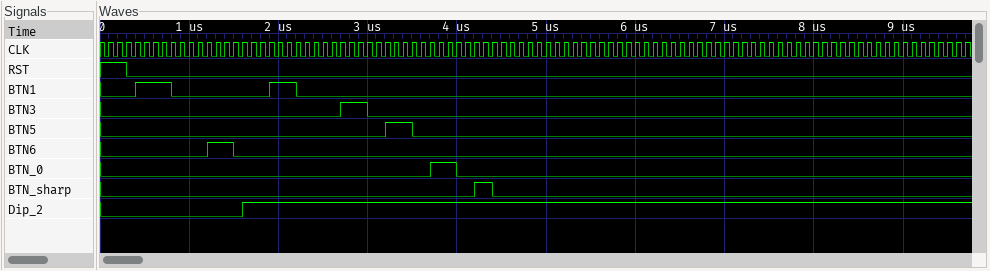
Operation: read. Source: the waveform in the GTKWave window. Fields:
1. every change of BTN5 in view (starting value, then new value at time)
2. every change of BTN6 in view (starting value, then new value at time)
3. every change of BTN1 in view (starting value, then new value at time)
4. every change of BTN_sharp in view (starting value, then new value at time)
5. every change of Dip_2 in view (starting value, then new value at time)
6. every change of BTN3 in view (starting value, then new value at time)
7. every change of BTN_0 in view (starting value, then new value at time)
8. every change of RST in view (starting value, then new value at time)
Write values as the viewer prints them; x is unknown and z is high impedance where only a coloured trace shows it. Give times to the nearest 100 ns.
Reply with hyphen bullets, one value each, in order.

- 0, 1 at 3200 ns, 0 at 3500 ns
- 0, 1 at 1200 ns, 0 at 1500 ns
- 0, 1 at 400 ns, 0 at 800 ns, 1 at 1900 ns, 0 at 2200 ns
- 0, 1 at 4200 ns, 0 at 4400 ns
- 0, 1 at 1600 ns
- 0, 1 at 2700 ns, 0 at 3000 ns
- 0, 1 at 3700 ns, 0 at 4000 ns
- 1, 0 at 300 ns
